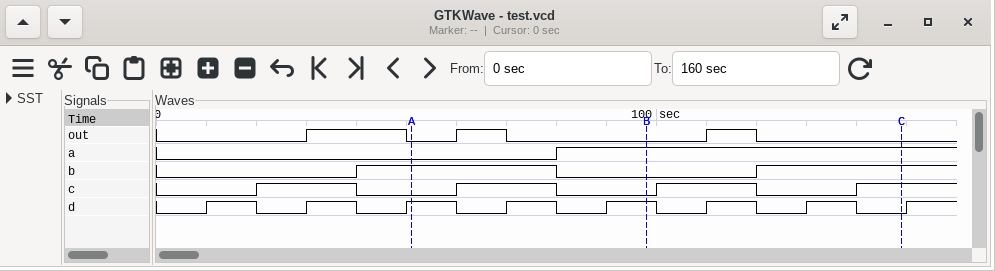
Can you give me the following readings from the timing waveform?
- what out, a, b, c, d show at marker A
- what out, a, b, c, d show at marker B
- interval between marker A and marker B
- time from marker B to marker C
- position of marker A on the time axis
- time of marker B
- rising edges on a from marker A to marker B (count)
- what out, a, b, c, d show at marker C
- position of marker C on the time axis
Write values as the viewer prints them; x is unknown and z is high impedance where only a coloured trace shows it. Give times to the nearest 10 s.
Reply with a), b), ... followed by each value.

a) out=0, a=0, b=1, c=0, d=1
b) out=0, a=1, b=0, c=0, d=1
c) 50 s
d) 50 s
e) 50 s
f) 100 s
g) 1
h) out=0, a=1, b=1, c=1, d=0
i) 150 s
